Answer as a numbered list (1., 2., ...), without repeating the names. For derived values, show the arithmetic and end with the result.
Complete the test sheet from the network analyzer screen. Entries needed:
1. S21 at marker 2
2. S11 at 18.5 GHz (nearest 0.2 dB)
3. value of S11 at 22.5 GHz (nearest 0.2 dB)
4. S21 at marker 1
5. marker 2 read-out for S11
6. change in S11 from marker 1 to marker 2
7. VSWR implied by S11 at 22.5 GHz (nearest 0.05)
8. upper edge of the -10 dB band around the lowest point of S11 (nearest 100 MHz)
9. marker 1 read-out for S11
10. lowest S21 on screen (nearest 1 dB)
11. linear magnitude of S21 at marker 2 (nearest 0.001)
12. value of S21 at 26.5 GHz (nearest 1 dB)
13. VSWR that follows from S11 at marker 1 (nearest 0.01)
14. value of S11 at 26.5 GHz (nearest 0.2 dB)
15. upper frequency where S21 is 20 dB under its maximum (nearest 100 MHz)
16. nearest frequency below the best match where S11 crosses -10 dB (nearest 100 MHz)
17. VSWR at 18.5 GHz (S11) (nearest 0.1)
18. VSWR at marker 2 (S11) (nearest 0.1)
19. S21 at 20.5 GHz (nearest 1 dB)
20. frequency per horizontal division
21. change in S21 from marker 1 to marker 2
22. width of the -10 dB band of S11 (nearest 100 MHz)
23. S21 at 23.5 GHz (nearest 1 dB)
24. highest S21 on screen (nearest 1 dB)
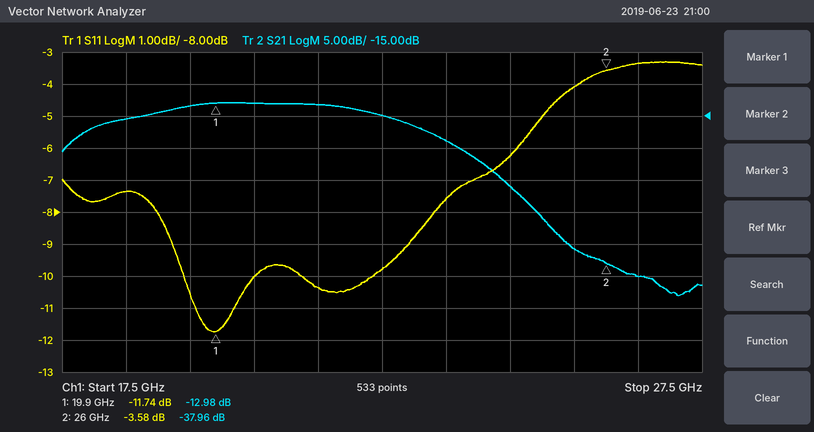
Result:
1. -37.96 dB
2. -7.4 dB
3. -9.8 dB
4. -12.98 dB
5. -3.58 dB
6. -3.58 − (-11.74) = 8.16 dB
7. |Γ| = 10^(-9.8/20) = 0.3236; VSWR = (1 + 0.3236)/(1 − 0.3236) ≈ 1.96, so 1.95 to the nearest 0.05
8. 20.5 GHz
9. -11.74 dB
10. -43 dB
11. 10^(-37.96/20) ≈ 0.013
12. -40 dB
13. (1 + 0.2588)/(1 − 0.2588) ≈ 1.70
14. -3.4 dB
15. 25.2 GHz
16. 19.4 GHz
17. |Γ| = 10^(-7.4/20) = 0.4266; VSWR = (1 + 0.4266)/(1 − 0.4266) ≈ 2.5
18. (1 + 0.6622)/(1 − 0.6622) ≈ 4.9
19. -13 dB
20. 1 GHz
21. -37.96 − (-12.98) = -24.98 dB
22. 20.5 GHz − 19.4 GHz = 1.1 GHz
23. -19 dB
24. -13 dB
